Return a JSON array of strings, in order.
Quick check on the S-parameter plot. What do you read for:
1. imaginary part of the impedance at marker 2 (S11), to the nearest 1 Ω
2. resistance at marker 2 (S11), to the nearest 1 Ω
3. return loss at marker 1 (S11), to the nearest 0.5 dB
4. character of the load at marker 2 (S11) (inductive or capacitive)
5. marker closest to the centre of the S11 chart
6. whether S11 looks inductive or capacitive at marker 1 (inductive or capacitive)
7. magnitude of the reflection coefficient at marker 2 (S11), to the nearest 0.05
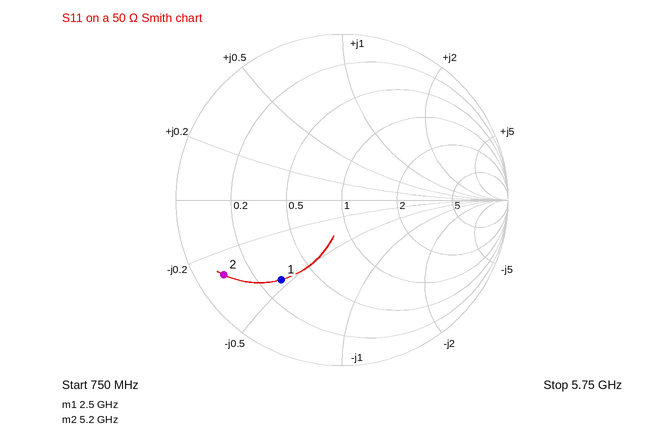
["-14 Ω", "5 Ω", "4.5 dB", "capacitive", "marker 1", "capacitive", "0.85"]
